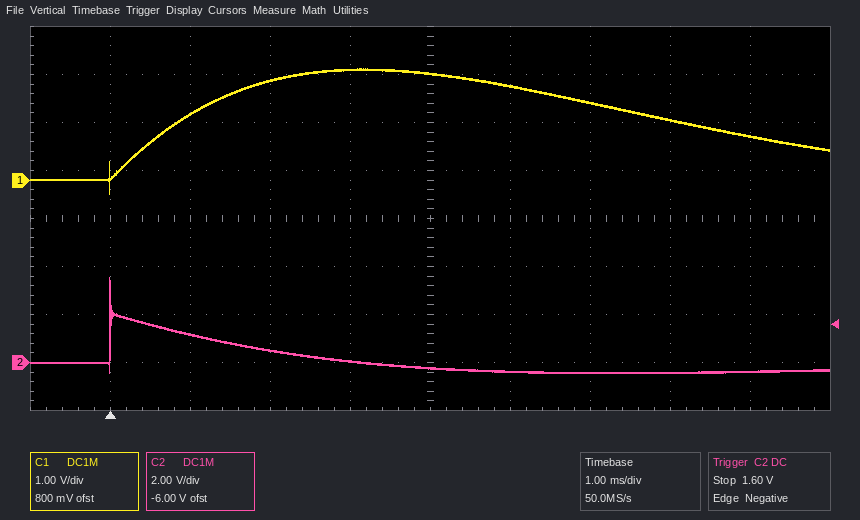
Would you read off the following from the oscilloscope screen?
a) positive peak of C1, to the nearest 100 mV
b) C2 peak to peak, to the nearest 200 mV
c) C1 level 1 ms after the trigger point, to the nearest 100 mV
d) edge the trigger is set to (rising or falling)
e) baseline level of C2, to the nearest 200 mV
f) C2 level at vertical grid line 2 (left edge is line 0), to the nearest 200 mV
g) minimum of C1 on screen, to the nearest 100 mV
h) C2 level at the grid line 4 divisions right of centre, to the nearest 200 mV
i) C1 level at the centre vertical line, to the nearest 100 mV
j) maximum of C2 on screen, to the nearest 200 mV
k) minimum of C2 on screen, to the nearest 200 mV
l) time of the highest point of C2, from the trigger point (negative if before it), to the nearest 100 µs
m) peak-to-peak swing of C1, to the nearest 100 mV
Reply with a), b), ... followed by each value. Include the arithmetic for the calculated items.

a) 2.3 V
b) 3.6 V − (-400 mV) = 4.0 V
c) 1.4 V
d) falling
e) -400 mV
f) 1.2 V
g) -300 mV
h) -400 mV
i) 2.2 V
j) 3.6 V
k) -400 mV
l) 0.0 ms
m) 2.3 V − (-300 mV) = 2.6 V
